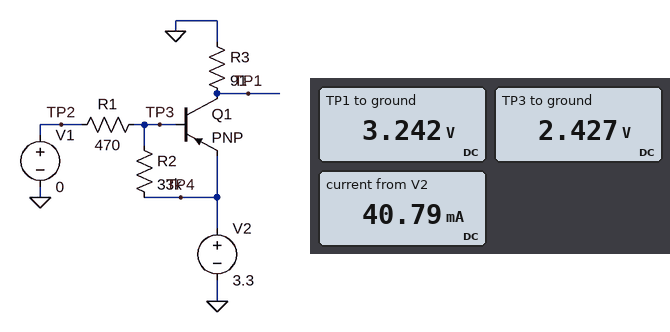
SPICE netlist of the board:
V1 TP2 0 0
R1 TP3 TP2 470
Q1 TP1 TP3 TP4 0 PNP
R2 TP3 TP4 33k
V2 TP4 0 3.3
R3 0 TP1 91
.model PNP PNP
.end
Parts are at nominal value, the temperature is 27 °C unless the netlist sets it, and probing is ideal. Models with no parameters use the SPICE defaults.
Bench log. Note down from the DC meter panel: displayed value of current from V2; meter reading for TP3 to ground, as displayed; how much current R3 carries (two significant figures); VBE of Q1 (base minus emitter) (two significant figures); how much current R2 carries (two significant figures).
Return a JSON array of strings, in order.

["40.79 mA", "2.427 V", "36 mA", "-870 mV", "26 µA"]
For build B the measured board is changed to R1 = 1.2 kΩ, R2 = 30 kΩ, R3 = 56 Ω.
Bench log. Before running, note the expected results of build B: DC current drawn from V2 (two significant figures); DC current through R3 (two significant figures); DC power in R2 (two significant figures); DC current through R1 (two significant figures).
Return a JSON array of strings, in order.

["59 mA", "57 mA", "26 µW", "2.0 mA"]
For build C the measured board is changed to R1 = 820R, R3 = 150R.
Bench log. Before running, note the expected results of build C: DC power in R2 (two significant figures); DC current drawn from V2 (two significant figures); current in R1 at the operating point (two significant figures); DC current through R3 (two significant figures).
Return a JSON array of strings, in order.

["22 µW", "25 mA", "3.0 mA", "22 mA"]
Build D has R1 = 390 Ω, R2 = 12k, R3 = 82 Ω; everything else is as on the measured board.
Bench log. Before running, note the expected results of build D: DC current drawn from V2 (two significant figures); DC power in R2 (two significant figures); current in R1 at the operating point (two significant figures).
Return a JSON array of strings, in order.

["46 mA", "64 µW", "6.2 mA"]
